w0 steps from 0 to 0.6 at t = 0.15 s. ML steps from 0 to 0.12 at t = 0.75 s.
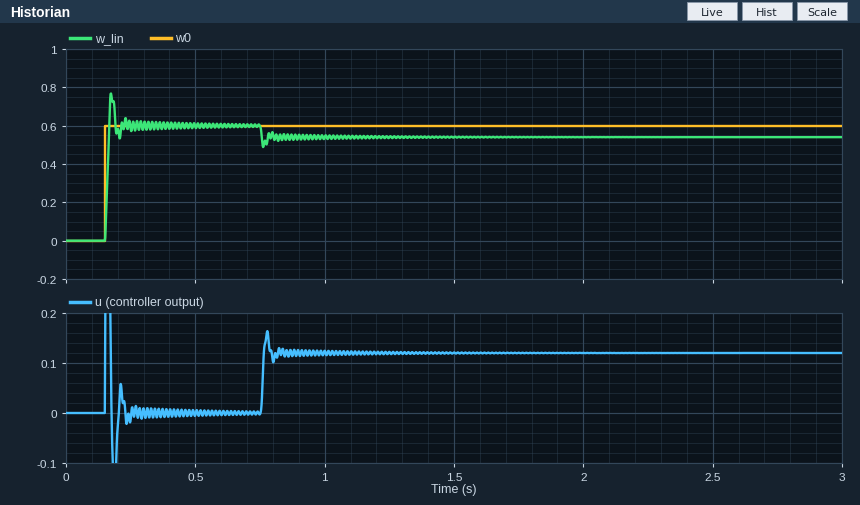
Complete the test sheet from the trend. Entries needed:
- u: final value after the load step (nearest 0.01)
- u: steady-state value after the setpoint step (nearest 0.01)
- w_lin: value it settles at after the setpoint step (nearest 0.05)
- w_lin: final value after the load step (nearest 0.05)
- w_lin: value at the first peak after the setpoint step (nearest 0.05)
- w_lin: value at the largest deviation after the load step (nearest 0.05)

0.12
0.00
0.60
0.55
0.75
0.50
